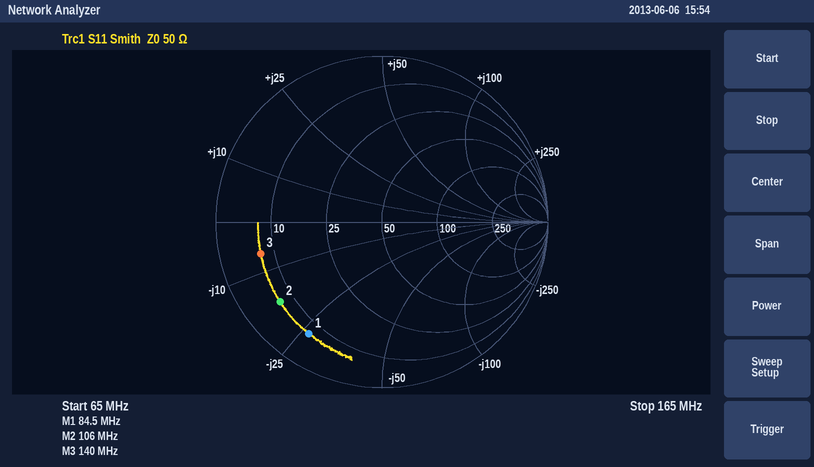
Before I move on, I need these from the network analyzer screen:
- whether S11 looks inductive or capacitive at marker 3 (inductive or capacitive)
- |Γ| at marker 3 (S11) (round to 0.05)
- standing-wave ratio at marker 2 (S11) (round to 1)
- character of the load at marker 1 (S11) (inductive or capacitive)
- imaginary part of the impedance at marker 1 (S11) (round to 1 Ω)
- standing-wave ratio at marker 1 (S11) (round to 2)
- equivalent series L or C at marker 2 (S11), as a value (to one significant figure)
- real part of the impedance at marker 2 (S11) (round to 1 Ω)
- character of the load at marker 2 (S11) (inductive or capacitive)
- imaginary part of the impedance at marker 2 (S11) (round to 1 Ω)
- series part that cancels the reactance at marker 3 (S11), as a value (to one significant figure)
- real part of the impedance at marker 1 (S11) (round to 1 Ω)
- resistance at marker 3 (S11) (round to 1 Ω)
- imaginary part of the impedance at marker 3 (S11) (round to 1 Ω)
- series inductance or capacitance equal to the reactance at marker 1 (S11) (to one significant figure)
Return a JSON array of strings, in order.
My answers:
["capacitive", "0.75", "8", "capacitive", "-27 Ω", "10", "90 pF", "7 Ω", "capacitive", "-17 Ω", "7 nH", "7 Ω", "7 Ω", "-6 Ω", "70 pF"]
